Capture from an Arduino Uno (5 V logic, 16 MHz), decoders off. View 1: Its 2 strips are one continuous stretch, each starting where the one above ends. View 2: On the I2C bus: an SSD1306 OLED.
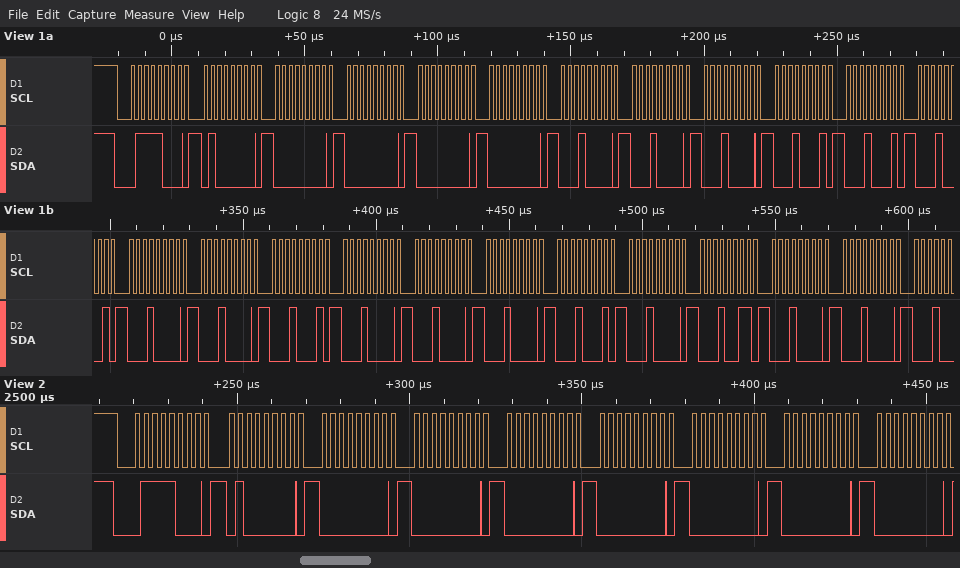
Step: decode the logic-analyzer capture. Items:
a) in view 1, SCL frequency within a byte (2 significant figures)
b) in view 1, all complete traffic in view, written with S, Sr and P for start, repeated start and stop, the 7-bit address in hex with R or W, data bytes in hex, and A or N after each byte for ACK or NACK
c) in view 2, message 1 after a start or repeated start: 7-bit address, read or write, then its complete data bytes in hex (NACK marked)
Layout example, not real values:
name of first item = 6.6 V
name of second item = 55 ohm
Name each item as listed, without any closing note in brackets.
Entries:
in view 1, SCL frequency within a byte = 400 kHz
in view 1, all complete traffic in view, written with S, Sr and P for start, repeated start and stop, the 7-bit address in hex with R or W, data bytes in hex, and A or N after each byte for ACK or NACK = S 3CW A 40 A 00 A 00 A 00 A 00 A 10 A 10 A 10 A 11 A 11 A 11 A 10 A 10 A 11 A 10 A 10 A 10 A 11 A 10 A 13 A 10 A 10 A
in view 2, message 1 after a start or repeated start: 7-bit address, read or write, then its complete data bytes in hex = 0x3C write: 40 00 00 00 00 00 00 00
